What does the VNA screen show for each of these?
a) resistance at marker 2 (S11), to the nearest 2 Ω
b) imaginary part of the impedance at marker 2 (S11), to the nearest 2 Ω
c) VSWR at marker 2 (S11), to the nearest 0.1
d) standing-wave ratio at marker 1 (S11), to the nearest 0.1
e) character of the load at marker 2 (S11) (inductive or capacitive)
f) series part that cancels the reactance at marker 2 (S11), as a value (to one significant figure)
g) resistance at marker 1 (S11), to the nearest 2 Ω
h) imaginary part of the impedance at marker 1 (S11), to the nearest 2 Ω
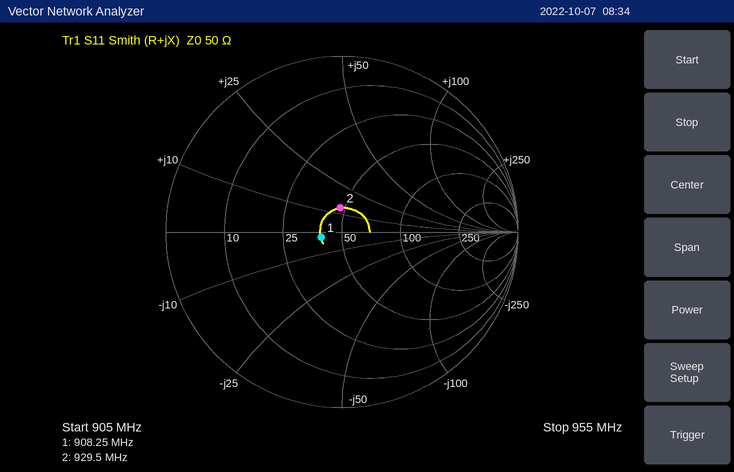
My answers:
48 Ω
+14 Ω
1.3
1.3
inductive
10 pF
40 Ω
-2 Ω
